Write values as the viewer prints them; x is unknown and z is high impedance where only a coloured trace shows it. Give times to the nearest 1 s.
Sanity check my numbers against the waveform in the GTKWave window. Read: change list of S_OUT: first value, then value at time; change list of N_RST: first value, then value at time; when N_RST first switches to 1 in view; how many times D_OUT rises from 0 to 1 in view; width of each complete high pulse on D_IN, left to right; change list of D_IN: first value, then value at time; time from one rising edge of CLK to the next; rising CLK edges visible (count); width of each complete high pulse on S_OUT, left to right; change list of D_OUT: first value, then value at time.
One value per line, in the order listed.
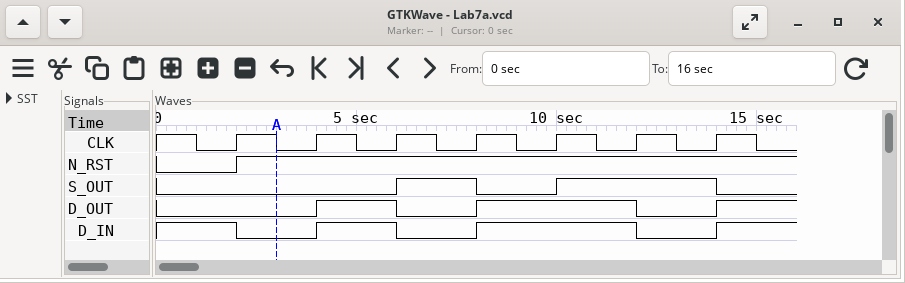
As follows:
0, 1 at 6 s, 0 at 8 s, 1 at 10 s, 0 at 14 s
0, 1 at 2 s
2 s
3
2 s, 4 s
1, 0 at 2 s, 1 at 4 s, 0 at 6 s, 1 at 8 s, 0 at 12 s, 1 at 14 s
2 s
7
2 s, 4 s
0, 1 at 4 s, 0 at 6 s, 1 at 8 s, 0 at 12 s, 1 at 14 s
